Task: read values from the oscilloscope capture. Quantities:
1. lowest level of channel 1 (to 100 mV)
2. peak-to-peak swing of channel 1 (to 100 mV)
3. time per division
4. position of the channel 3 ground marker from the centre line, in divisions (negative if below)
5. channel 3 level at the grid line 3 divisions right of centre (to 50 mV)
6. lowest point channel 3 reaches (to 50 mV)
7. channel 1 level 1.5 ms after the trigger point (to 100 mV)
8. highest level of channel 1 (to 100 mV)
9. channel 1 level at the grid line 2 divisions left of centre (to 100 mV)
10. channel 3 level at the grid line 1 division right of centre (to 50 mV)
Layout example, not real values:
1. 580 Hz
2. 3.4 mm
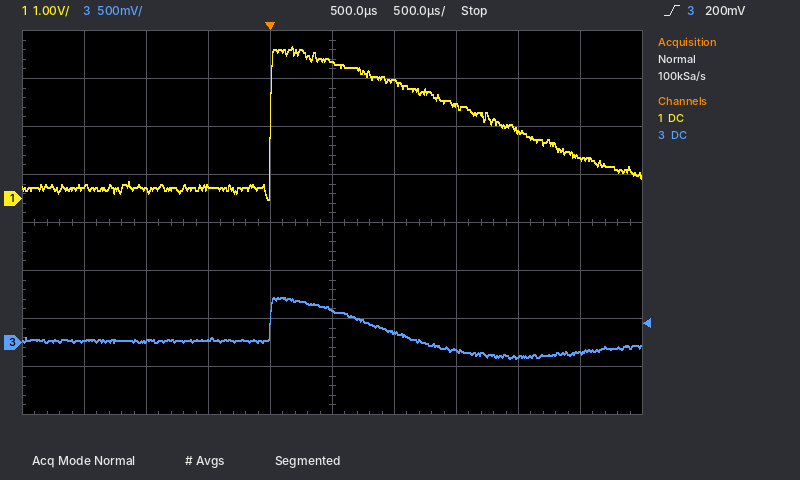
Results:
1. 0.0 V
2. 3.2 V
3. 500 µs
4. -2.5 div
5. -150 mV
6. -150 mV
7. 1.9 V
8. 3.2 V
9. 200 mV
10. 100 mV
